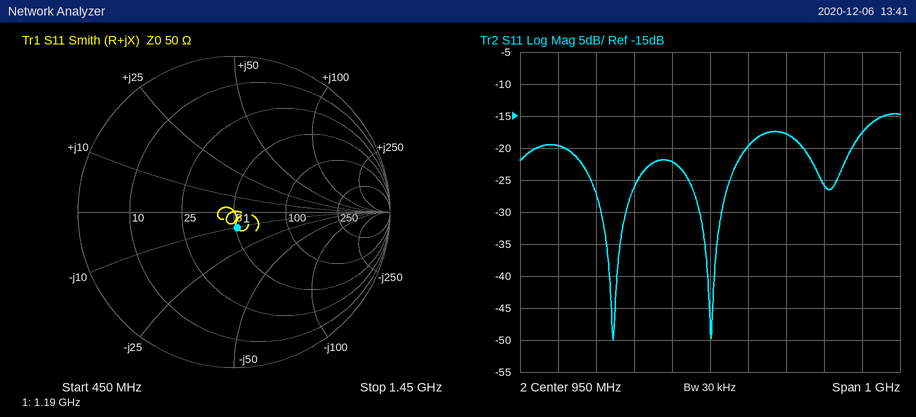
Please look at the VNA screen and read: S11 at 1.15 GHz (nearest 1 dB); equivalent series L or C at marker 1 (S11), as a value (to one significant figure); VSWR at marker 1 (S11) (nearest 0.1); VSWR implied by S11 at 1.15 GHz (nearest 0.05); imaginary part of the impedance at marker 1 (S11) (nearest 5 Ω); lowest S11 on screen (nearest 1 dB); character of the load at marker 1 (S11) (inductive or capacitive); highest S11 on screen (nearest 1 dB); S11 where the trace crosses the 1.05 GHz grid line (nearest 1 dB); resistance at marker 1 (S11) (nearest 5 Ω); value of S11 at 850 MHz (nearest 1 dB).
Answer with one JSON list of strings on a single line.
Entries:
["-18 dB", "10 pF", "1.2", "1.30", "-10 Ω", "-50 dB", "capacitive", "-15 dB", "-20 dB", "50 Ω", "-22 dB"]
